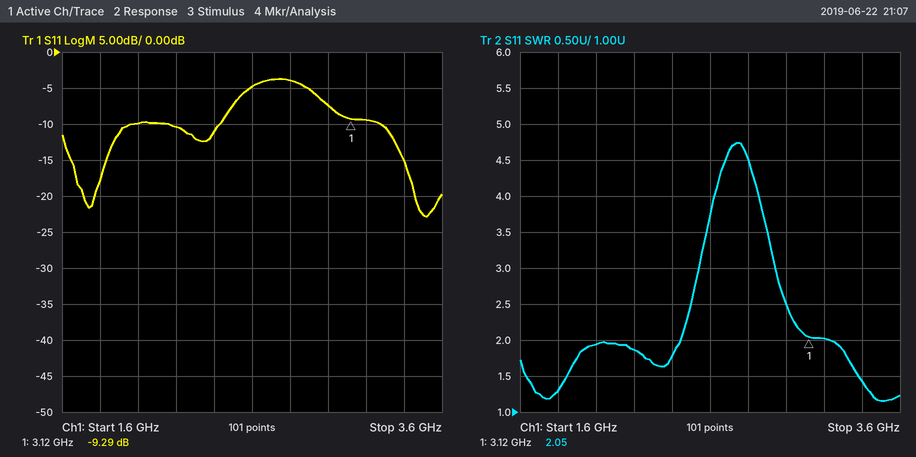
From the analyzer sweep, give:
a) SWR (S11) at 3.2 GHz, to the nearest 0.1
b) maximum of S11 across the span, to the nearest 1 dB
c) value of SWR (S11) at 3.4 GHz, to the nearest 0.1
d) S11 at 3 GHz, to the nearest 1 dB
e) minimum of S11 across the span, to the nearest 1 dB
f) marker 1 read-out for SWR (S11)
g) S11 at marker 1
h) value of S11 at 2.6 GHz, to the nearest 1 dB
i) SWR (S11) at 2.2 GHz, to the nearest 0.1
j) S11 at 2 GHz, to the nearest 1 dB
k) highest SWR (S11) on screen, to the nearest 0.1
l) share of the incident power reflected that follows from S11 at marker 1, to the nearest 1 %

2.0
-4 dB
1.4
-7 dB
-23 dB
2.05
-9.29 dB
-5 dB
1.9
-10 dB
4.7
12 %
